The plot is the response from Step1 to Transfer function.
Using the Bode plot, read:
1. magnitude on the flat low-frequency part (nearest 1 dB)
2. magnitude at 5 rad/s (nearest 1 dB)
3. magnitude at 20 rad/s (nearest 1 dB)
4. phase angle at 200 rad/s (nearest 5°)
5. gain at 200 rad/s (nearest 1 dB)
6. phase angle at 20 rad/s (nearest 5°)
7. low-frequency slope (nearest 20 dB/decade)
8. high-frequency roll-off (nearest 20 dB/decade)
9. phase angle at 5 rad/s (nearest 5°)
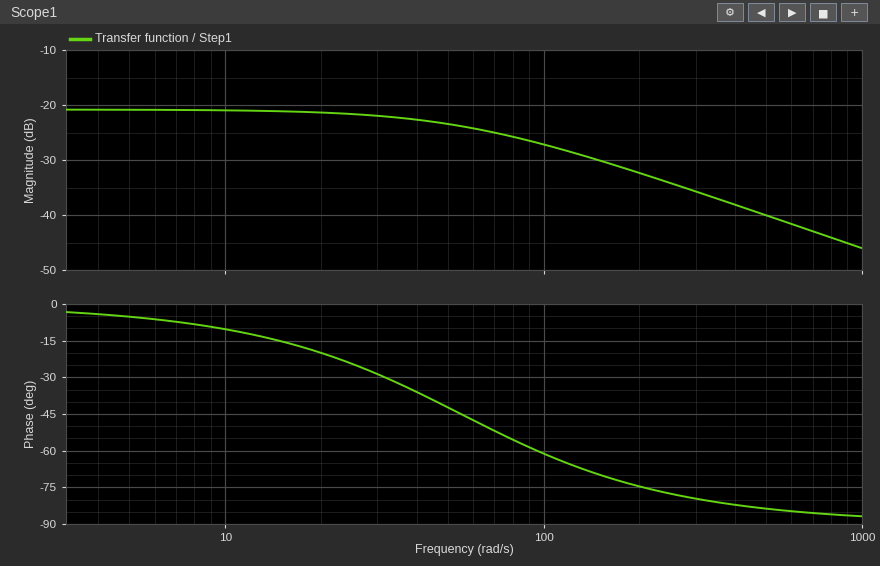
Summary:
-21 dB
-21 dB
-21 dB
-75°
-32 dB
-20°
0 dB/decade
-20 dB/decade
-5°
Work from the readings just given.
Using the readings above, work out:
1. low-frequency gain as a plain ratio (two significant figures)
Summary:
0.089
